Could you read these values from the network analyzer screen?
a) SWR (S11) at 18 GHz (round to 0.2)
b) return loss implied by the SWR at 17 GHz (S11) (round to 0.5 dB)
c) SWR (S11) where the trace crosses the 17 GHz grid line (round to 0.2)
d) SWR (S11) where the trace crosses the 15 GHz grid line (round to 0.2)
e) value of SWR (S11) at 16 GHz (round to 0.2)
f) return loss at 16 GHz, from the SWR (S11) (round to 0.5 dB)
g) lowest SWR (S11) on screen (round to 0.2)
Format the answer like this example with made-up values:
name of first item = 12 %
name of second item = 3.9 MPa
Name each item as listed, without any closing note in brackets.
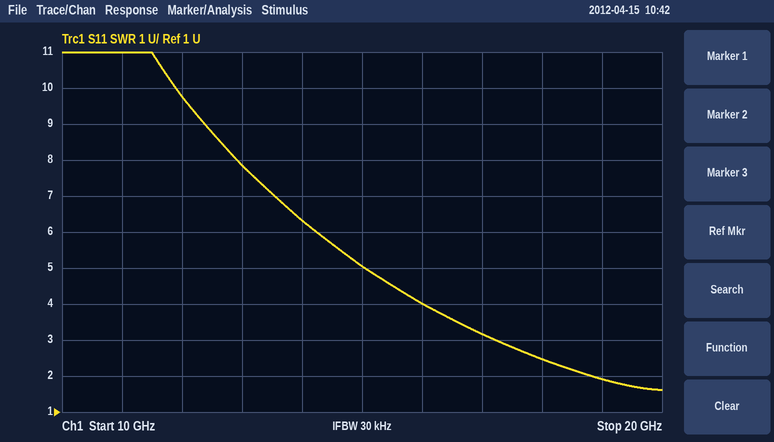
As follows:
SWR (S11) at 18 GHz = 2.4
return loss implied by the SWR at 17 GHz (S11) = 5.5 dB
SWR (S11) where the trace crosses the 17 GHz grid line = 3.2
SWR (S11) where the trace crosses the 15 GHz grid line = 5.0
value of SWR (S11) at 16 GHz = 4.0
return loss at 16 GHz, from the SWR (S11) = 4.5 dB
lowest SWR (S11) on screen = 1.6
